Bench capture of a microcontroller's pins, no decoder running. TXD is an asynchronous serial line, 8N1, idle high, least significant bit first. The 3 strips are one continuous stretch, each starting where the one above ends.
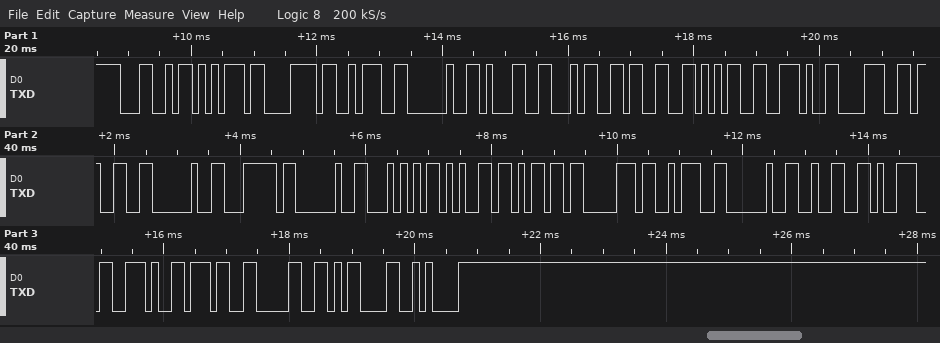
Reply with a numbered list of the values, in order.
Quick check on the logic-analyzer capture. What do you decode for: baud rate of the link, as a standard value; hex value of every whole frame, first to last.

1. 9600 baud
2. 0x4C 0x75 0x78 0x3A 0x20 0x31 0x34 0x33 0x35 0x2E 0x38 0x33 0x20 0x7C 0x20 0x54 0x65 0x6D 0x70 0x3A 0x20 0x32 0x39 0x2E 0x37 0x30 0x0D 0x0A
